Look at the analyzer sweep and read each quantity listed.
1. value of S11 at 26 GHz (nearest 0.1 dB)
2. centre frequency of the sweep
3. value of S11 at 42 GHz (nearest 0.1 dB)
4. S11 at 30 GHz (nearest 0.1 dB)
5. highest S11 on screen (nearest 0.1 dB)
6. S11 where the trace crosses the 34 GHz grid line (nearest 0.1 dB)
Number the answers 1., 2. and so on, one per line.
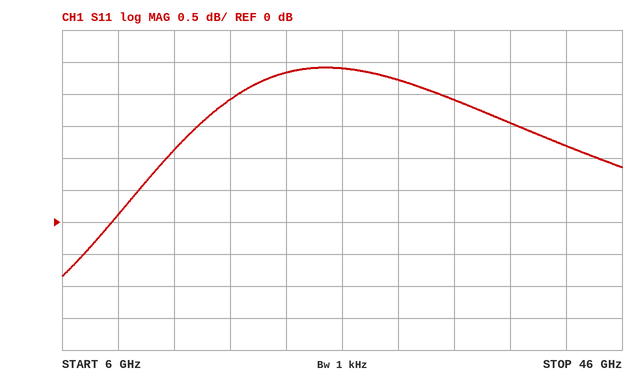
1. 2.4 dB
2. 26 GHz
3. 1.2 dB
4. 2.2 dB
5. 2.4 dB
6. 1.9 dB
